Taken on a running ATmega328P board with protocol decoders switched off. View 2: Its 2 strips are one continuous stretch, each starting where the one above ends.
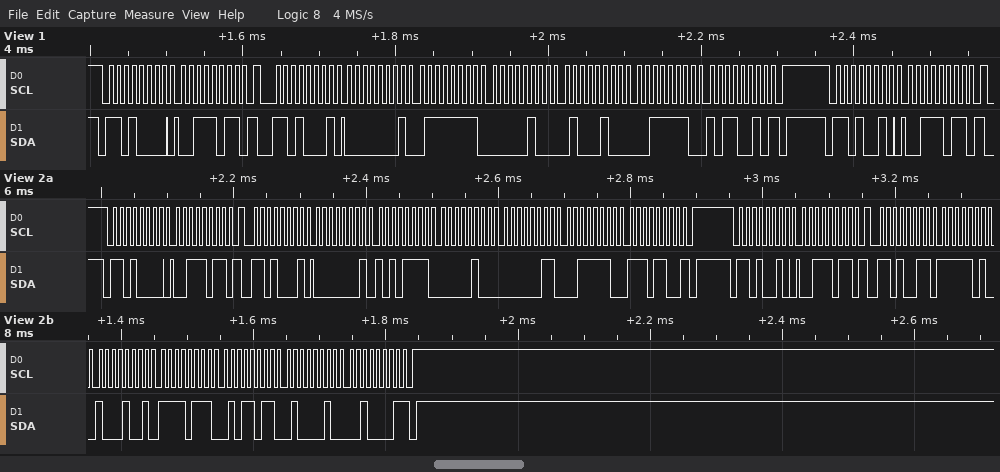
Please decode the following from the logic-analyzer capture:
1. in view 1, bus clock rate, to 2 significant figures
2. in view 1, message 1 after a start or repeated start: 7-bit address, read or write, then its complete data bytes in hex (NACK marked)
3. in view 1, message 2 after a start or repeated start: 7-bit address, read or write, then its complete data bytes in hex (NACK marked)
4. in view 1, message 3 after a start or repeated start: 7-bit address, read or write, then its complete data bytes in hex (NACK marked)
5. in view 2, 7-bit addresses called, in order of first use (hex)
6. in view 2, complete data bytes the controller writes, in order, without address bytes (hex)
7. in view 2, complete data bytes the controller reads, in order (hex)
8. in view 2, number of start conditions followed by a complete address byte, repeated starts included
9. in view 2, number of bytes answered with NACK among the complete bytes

100 kHz
0x68 write: 3B
0x68 read: 01 7F 04 44 3E B2 NACK
0x69 write: 3B
0x68 0x69
3B 3B
01 AF 04 03 3E EC FA 89 F7 5B 42 21
4
2
